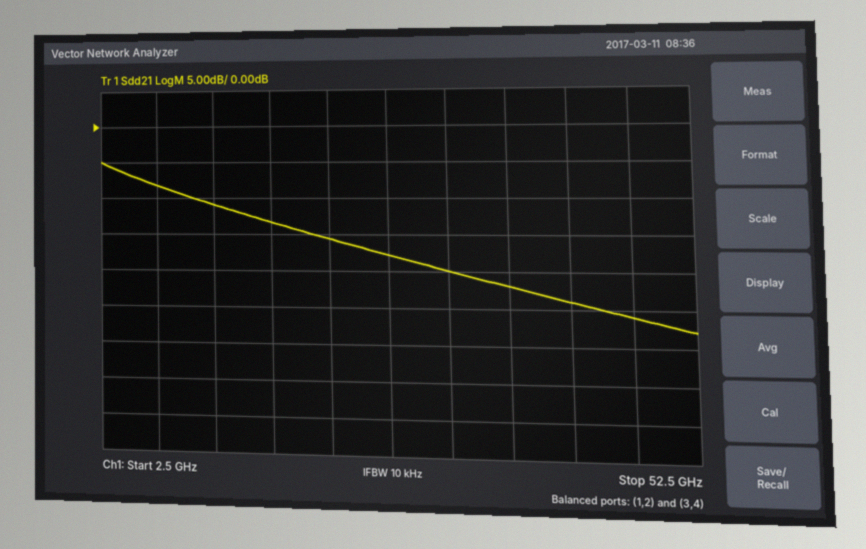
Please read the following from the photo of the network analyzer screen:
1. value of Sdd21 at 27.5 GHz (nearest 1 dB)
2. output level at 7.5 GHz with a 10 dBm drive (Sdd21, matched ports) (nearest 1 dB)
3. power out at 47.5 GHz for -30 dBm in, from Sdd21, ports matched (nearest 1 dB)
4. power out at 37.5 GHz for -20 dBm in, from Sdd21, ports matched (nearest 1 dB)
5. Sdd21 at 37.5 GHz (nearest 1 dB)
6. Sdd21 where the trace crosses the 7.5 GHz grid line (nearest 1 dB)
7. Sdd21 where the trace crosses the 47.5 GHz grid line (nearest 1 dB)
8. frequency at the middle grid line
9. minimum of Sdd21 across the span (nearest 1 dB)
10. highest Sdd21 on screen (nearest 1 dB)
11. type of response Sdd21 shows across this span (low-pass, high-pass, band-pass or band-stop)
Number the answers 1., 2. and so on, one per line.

1. -18 dB
2. 2 dBm
3. -56 dBm
4. -42 dBm
5. -22 dB
6. -8 dB
7. -26 dB
8. 27.5 GHz
9. -28 dB
10. -5 dB
11. low-pass
